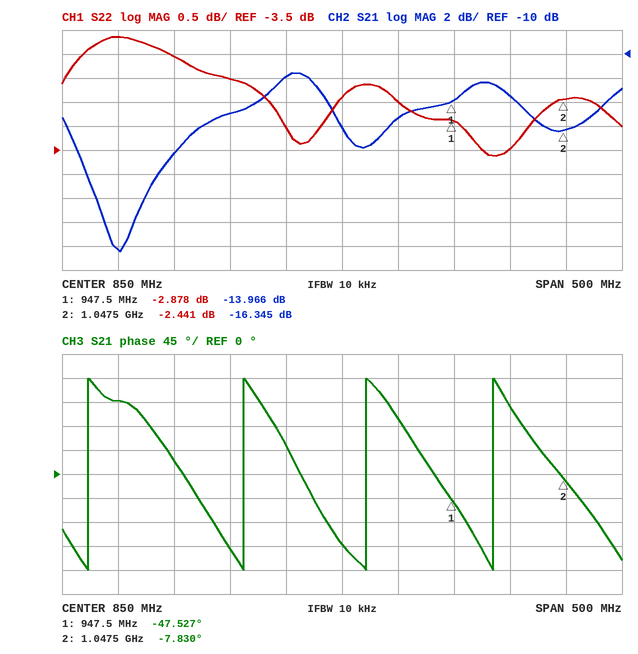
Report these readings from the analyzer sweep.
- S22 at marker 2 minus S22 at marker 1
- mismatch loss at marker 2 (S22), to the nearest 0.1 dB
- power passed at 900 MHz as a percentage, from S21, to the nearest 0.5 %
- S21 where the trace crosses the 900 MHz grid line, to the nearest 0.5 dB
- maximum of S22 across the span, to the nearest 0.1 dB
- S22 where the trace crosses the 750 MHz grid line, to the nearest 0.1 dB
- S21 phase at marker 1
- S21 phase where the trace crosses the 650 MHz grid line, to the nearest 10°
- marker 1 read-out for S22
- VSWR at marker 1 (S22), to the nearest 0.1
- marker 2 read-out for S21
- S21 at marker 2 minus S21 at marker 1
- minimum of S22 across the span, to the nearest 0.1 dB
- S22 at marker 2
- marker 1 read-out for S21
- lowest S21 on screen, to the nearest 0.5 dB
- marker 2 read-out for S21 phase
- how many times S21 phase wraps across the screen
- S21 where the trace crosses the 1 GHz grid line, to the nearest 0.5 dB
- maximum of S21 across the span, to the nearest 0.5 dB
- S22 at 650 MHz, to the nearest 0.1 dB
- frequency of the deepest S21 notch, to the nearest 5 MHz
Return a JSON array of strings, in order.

["0.437 dB", "3.7 dB", "3.0 %", "-15.5 dB", "-1.1 dB", "-2.0 dB", "-47.527°", "140°", "-2.878 dB", "6.1", "-16.345 dB", "-2.379 dB", "-3.6 dB", "-2.441 dB", "-13.966 dB", "-26.5 dB", "-7.830°", "4", "-13.5 dB", "-11.5 dB", "-1.1 dB", "650 MHz"]
